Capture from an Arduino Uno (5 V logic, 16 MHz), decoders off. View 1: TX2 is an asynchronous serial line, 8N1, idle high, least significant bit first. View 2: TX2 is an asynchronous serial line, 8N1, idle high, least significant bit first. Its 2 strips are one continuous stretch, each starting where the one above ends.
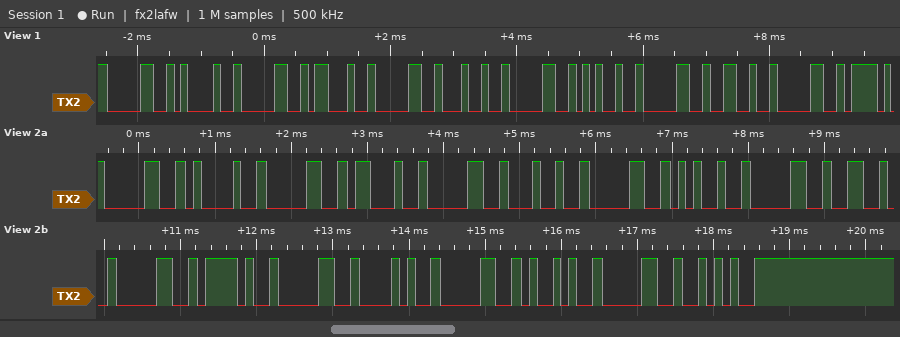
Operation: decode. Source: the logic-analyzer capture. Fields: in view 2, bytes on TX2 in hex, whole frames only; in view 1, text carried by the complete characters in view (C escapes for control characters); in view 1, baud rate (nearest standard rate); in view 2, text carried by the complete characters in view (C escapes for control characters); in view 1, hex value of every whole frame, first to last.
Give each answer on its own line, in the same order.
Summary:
0x30 0x21 0x30 0x23 0x30 0x24 0x30 0x25 0x30 0x26 0x30 0x2F 0x30 0x28 0x30 0x29 0x30 0x2A
"0!0#0$0%0&0"
9600 baud
"0!0#0$0%0&0/0(0)0*"
30 21 30 23 30 24 30 25 30 26 30
